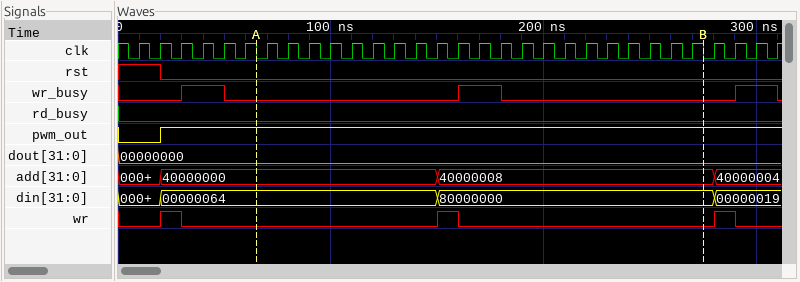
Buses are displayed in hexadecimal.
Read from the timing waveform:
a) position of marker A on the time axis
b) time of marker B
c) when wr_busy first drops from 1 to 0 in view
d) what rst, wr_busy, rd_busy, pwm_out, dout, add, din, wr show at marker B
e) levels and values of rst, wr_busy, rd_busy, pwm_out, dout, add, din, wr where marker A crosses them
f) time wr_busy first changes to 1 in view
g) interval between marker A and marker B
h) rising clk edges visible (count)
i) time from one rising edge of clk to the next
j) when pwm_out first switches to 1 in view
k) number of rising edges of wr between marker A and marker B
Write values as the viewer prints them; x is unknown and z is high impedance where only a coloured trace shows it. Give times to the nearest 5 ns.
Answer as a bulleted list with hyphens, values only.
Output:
- 65 ns
- 275 ns
- 50 ns
- rst=0, wr_busy=0, rd_busy=0, pwm_out=1, dout=00000000, add=40000008, din=80000000, wr=0
- rst=0, wr_busy=0, rd_busy=0, pwm_out=1, dout=00000000, add=40000000, din=00000064, wr=0
- 30 ns
- 210 ns
- 31
- 10 ns
- 20 ns
- 1
